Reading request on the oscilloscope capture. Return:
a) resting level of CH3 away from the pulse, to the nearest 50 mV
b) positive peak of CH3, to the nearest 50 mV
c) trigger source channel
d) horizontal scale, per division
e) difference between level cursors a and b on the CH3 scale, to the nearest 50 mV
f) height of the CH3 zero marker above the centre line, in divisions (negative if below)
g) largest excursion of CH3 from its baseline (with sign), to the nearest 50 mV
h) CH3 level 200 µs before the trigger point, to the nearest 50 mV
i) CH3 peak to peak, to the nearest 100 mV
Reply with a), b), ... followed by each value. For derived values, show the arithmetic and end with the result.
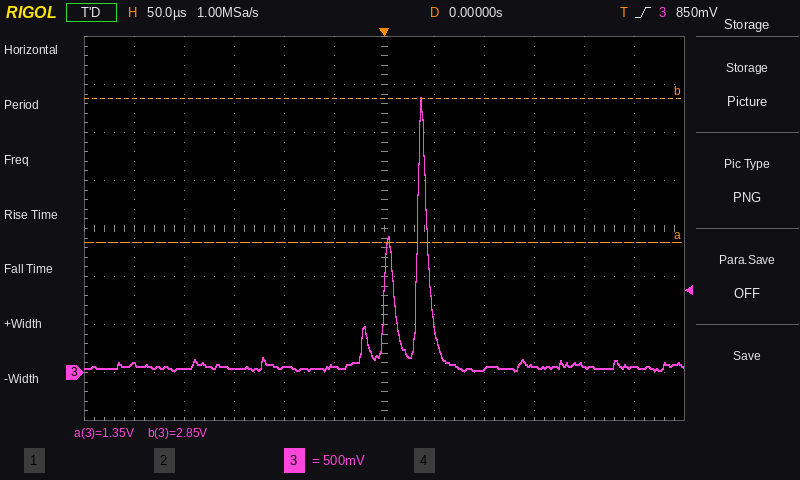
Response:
a) 50 mV
b) 2.85 V
c) CH3
d) 50 µs
e) 1.50 V
f) -3.0 div
g) 2.85 V − (50 mV) = +2.80 V
h) 50 mV
i) 2.80 V
